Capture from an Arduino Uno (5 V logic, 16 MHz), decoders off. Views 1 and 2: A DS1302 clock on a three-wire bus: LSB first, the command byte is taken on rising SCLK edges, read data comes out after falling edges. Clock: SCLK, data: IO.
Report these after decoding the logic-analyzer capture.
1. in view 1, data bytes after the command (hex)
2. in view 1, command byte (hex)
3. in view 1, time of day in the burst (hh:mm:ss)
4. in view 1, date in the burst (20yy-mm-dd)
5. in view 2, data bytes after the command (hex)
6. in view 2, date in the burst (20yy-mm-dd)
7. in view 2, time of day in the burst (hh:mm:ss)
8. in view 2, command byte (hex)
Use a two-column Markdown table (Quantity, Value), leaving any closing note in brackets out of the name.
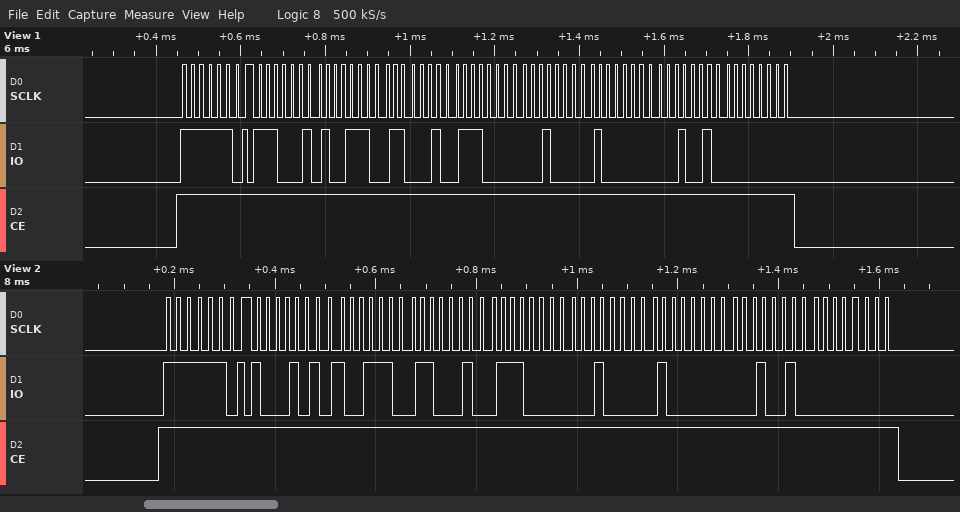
| Quantity | Value |
|---|---|
| in view 1, data bytes after the command | 47 39 23 07 04 01 24 00 |
| in view 1, command byte | 0xBF |
| in view 1, time of day in the burst | 23:39:47 |
| in view 1, date in the burst | 2024-04-07 |
| in view 2, data bytes after the command | 51 39 23 07 04 01 24 00 |
| in view 2, date in the burst | 2024-04-07 |
| in view 2, time of day in the burst | 23:39:51 |
| in view 2, command byte | 0xBF |
